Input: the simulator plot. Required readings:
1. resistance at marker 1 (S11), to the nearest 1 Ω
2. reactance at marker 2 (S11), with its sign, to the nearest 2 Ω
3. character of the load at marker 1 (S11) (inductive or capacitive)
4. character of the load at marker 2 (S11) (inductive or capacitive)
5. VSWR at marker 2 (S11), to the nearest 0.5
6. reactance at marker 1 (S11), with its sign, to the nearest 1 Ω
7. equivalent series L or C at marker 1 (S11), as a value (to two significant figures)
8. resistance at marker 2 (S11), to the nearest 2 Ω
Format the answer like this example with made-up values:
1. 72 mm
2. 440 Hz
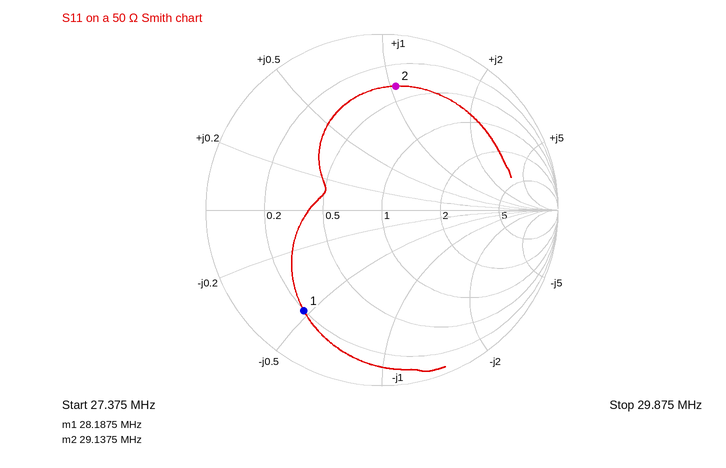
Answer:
1. 10 Ω
2. +52 Ω
3. capacitive
4. inductive
5. 6.0
6. -24 Ω
7. 240 pF
8. 18 Ω
